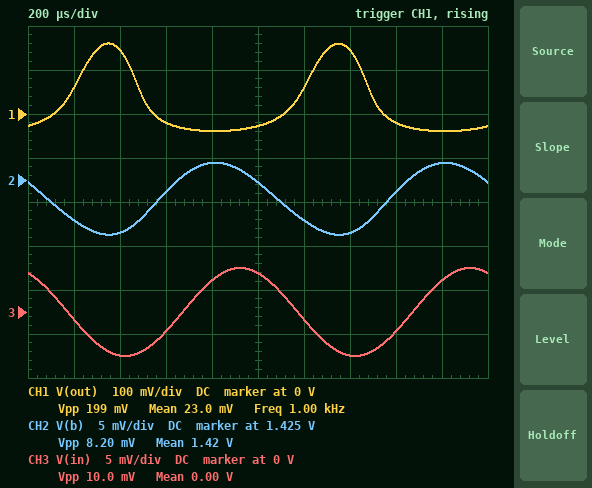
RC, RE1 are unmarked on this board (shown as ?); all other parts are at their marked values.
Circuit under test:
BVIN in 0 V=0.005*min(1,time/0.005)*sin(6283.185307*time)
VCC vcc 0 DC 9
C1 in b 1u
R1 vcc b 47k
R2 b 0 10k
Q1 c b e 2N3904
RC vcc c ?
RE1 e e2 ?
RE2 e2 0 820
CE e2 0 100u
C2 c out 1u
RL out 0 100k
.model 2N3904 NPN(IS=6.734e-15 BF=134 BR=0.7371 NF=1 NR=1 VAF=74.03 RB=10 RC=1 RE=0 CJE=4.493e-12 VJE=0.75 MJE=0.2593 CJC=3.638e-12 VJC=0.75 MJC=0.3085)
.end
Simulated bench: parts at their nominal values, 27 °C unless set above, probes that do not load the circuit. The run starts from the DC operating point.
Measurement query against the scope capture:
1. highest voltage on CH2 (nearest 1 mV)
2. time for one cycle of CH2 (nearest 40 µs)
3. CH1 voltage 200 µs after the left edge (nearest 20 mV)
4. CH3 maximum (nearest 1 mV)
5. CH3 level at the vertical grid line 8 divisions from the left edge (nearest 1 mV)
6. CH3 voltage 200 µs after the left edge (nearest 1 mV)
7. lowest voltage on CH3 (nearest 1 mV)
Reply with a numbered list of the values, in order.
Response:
1. 1.427 V
2. 1.00 ms
3. 60 mV
4. 5 mV
5. -2 mV
6. -1 mV
7. -5 mV
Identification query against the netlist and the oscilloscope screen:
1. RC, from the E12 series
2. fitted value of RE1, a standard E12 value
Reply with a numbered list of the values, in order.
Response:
1. 10 kΩ
2. 100 Ω
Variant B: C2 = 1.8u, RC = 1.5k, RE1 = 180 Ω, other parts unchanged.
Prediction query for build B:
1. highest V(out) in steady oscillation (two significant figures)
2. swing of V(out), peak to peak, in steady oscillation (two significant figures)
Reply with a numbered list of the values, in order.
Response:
1. 35 mV
2. 70 mV
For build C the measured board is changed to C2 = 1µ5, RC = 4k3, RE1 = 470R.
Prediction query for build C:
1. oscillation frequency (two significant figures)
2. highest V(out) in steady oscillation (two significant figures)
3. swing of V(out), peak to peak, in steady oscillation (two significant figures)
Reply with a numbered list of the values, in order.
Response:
1. 1.0 kHz
2. 40 mV
3. 80 mV
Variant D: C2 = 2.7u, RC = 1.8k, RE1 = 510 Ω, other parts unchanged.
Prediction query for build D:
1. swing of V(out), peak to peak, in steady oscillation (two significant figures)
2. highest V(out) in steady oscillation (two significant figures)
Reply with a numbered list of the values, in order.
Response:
1. 32 mV
2. 16 mV
